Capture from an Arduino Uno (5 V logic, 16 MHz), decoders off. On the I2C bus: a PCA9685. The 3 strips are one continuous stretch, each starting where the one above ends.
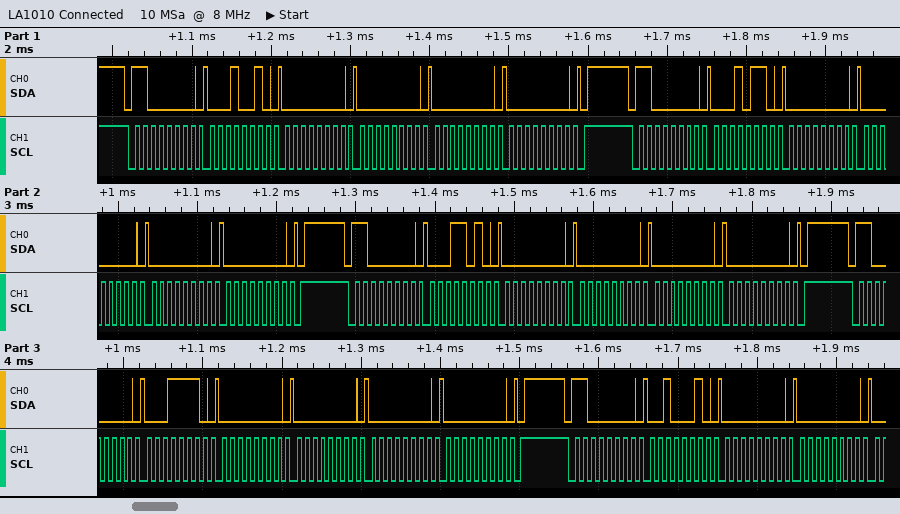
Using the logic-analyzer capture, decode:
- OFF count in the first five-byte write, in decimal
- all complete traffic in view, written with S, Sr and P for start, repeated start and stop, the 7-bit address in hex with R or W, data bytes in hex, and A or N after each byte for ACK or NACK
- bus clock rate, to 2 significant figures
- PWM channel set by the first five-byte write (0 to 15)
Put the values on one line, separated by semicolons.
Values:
0; S 60W A 12 A 00 A 00 A 00 A 00 A P S 60W A 16 A 00 A 00 A 00 A 00 A P S 60W A 1A A 00 A 00 A 00 A 00 A P S 60W A 1E A 00 A 00 A 00 A 00 A P S 60W A 22 A 00 A 00 A; 100 kHz; 3
